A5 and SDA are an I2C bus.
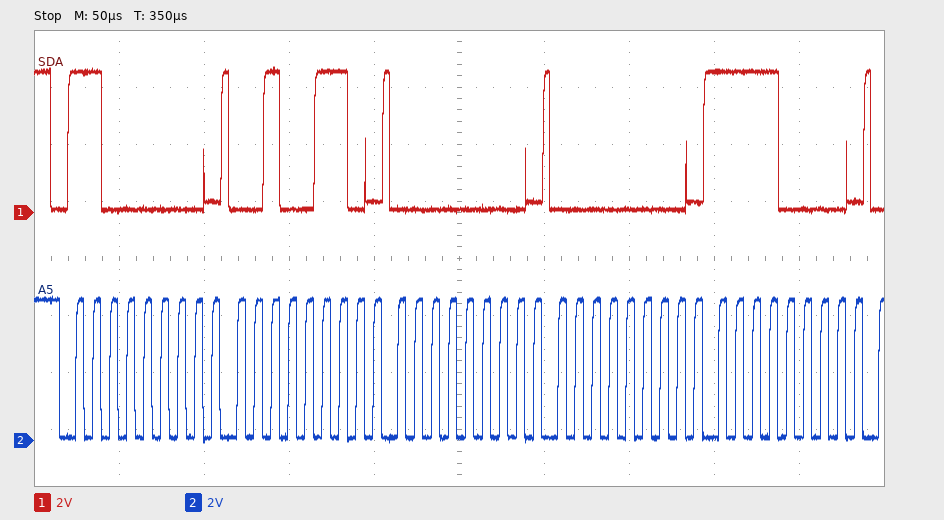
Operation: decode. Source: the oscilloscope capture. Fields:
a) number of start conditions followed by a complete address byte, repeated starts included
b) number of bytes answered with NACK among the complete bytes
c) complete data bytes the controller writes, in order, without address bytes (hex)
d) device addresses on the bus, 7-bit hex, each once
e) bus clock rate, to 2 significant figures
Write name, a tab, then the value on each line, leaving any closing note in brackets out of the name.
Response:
number of start conditions followed by a complete address byte, repeated starts included	1
number of bytes answered with NACK among the complete bytes	0
complete data bytes the controller writes, in order, without address bytes	26 00 00 F0
device addresses on the bus, 7-bit hex, each once	0x60
bus clock rate, to 2 significant figures	100 kHz
